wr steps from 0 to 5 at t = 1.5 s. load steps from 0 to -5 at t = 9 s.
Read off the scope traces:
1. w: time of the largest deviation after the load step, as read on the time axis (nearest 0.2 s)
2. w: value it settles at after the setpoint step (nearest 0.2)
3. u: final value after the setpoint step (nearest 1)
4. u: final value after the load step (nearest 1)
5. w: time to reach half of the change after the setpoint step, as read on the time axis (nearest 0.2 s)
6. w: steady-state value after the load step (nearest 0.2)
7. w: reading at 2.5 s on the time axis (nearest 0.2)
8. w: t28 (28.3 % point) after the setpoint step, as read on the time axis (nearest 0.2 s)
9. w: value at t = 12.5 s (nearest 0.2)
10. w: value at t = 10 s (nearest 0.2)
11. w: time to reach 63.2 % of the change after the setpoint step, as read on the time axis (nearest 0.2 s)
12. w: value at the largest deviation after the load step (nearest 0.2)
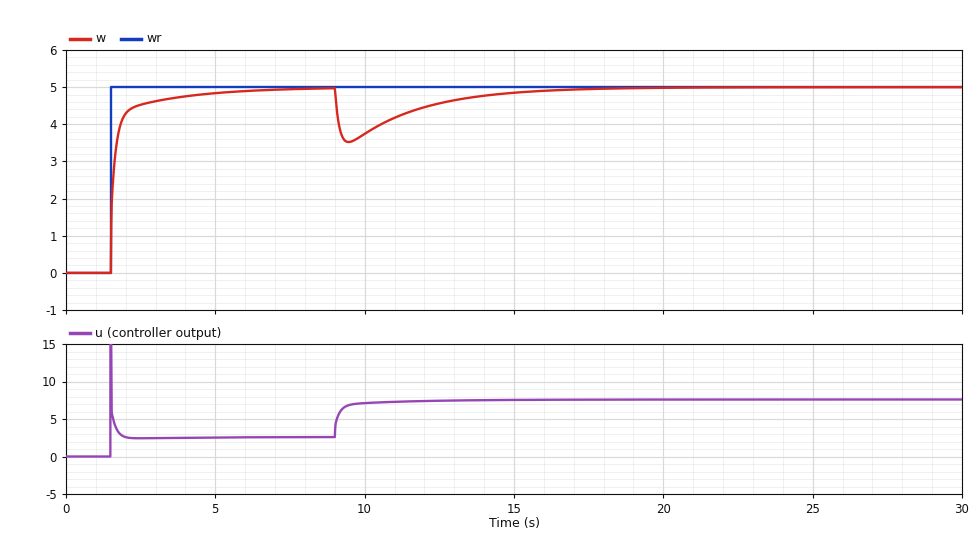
9.4 s
5.0
3
8
1.6 s
5.0
4.6
1.6 s
4.6
3.8
1.6 s
3.6
